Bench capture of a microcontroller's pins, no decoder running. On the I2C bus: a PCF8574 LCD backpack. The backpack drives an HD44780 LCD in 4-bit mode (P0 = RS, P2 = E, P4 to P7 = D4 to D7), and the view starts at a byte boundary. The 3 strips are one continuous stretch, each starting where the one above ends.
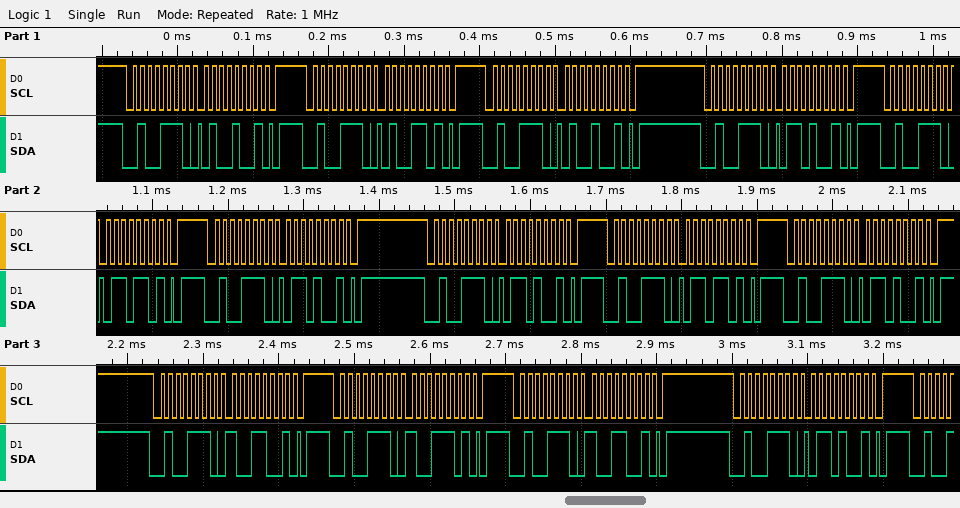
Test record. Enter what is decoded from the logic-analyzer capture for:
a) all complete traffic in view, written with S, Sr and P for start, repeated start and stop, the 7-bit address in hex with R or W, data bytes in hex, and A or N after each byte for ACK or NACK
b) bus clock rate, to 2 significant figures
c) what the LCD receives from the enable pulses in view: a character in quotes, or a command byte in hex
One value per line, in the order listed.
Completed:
S 27W A 49 A P S 27W A 4D A P S 27W A 49 A P S 27W A 69 A P S 27W A 6D A P S 27W A 69 A P S 27W A 69 A P S 27W A 6D A P S 27W A 69 A P S 27W A 99 A P S 27W A 9D A P S 27W A 99 A P S 27W A 69 A P
100 kHz
'F' 'i'
